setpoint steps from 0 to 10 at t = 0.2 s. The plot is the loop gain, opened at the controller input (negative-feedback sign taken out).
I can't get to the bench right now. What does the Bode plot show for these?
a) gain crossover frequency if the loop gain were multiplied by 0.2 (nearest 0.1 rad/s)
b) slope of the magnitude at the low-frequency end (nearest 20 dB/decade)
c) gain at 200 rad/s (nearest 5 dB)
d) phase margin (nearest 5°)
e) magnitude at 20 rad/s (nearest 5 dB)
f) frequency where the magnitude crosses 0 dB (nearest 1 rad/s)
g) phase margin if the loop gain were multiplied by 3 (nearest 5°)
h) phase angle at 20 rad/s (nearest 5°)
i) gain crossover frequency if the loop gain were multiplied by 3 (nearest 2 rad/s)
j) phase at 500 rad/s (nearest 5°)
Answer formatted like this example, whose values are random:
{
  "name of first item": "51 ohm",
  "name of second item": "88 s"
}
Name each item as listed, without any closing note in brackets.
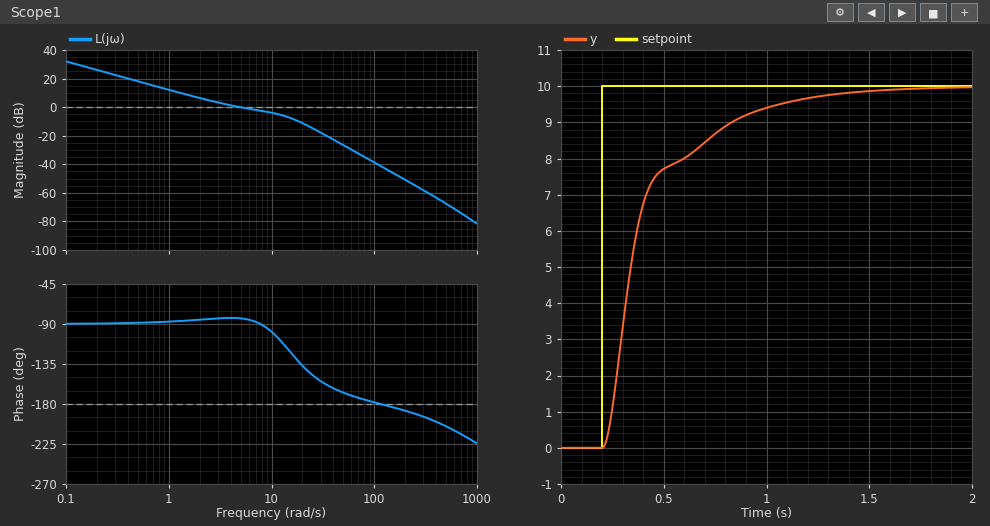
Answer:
{
  "gain crossover frequency if the loop gain were multiplied by 0.2": "0.8 rad/s",
  "slope of the magnitude at the low-frequency end": "-20 dB/decade",
  "gain at 200 rad/s": "-50 dB",
  "phase margin": "95°",
  "magnitude at 20 rad/s": "-10 dB",
  "frequency where the magnitude crosses 0 dB": "5 rad/s",
  "phase margin if the loop gain were multiplied by 3": "50°",
  "phase angle at 20 rad/s": "-135°",
  "gain crossover frequency if the loop gain were multiplied by 3": "18 rad/s",
  "phase at 500 rad/s": "-205°"
}
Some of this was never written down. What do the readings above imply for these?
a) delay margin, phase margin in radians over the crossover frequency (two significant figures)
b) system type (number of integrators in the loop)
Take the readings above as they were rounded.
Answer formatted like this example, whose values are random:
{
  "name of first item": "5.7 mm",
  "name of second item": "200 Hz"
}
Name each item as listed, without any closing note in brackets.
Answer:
{
  "delay margin, phase margin in radians over the crossover frequency": "0.33 s",
  "system type": "1"
}
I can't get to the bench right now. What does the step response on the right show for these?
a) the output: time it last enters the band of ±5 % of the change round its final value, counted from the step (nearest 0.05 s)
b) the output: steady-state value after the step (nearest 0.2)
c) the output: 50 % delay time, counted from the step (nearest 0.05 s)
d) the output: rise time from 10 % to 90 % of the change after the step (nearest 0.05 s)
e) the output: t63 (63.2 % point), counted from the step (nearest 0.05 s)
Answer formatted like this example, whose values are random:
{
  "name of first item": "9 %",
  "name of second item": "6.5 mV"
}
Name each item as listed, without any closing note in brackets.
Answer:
{
  "the output: time it last enters the band of ±5 % of the change round its final value, counted from the step": "0.85 s",
  "the output: steady-state value after the step": "10.0",
  "the output: 50 % delay time, counted from the step": "0.15 s",
  "the output: rise time from 10 % to 90 % of the change after the step": "0.60 s",
  "the output: t63 (63.2 % point), counted from the step": "0.20 s"
}
